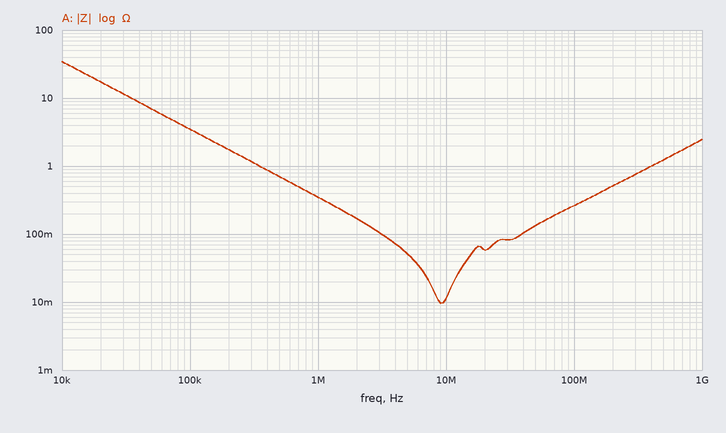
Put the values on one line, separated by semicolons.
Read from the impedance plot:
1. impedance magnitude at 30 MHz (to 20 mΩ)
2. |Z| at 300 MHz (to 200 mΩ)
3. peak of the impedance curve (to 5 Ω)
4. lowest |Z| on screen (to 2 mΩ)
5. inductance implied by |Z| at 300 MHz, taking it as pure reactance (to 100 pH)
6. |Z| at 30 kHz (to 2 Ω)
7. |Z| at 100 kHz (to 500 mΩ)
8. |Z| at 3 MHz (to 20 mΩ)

80 mΩ; 800 mΩ; 35 Ω; 10 mΩ; 400 pH; 12 Ω; 3.5 Ω; 100 mΩ
